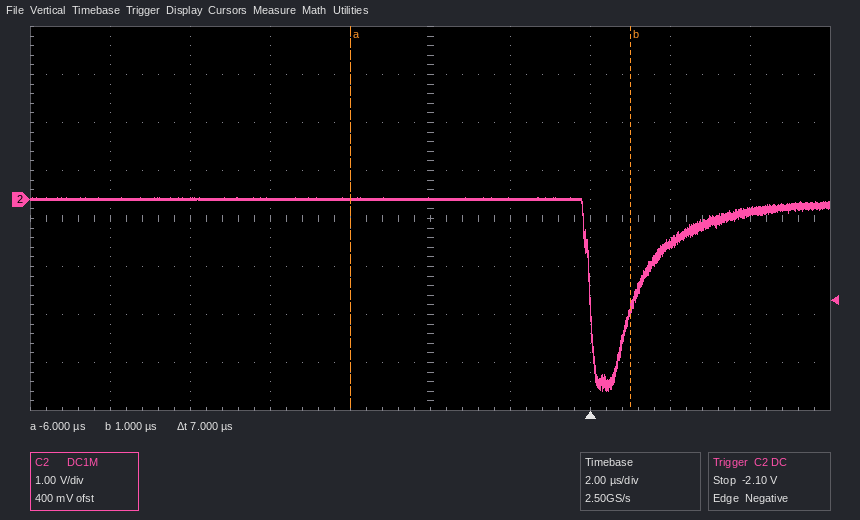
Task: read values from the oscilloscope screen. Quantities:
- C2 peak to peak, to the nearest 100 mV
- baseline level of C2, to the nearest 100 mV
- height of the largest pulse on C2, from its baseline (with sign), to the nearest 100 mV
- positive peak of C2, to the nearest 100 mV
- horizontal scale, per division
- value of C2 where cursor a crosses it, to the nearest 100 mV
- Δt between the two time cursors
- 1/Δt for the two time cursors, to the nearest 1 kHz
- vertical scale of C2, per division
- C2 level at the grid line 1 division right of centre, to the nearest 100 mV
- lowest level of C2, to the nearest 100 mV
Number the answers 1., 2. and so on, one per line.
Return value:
1. 4.0 V
2. 0.0 V
3. -4.0 V
4. 0.0 V
5. 2 µs
6. 0.0 V
7. 7 µs
8. 143 kHz
9. 1 V
10. 0.0 V
11. -4.0 V
